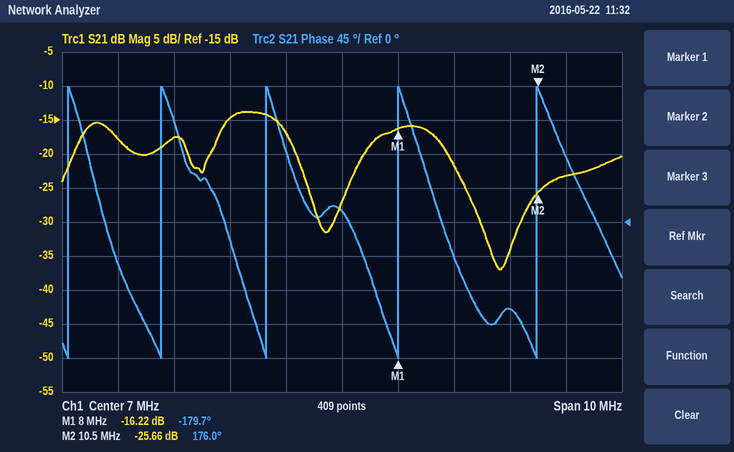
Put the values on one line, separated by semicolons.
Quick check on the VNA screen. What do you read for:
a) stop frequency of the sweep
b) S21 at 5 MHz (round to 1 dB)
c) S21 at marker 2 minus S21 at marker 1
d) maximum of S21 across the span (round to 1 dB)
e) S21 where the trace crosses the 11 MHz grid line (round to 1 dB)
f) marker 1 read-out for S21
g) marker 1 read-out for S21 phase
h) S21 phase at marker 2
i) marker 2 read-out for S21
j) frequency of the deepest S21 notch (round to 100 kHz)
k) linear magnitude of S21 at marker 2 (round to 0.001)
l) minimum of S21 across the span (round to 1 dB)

12 MHz; -15 dB; -9.44 dB; -14 dB; -23 dB; -16.22 dB; -179.7°; 176.0°; -25.66 dB; 9.8 MHz; 0.052; -37 dB
